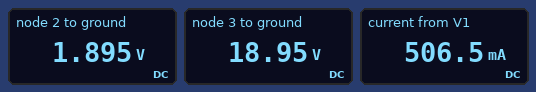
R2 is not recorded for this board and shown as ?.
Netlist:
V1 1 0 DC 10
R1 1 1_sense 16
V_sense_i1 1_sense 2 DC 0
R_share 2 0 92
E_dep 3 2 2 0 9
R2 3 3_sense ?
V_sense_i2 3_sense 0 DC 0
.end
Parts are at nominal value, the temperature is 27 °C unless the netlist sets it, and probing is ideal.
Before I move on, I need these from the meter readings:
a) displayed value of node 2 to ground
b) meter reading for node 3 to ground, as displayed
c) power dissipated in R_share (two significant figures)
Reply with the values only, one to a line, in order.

1.895 V
18.95 V
39 mW
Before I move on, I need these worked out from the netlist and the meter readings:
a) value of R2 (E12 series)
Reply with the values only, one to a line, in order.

39 Ω
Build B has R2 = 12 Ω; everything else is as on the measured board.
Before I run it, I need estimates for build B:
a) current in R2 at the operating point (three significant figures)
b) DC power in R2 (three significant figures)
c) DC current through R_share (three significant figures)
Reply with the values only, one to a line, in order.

574 mA
3.96 W
7.49 mA
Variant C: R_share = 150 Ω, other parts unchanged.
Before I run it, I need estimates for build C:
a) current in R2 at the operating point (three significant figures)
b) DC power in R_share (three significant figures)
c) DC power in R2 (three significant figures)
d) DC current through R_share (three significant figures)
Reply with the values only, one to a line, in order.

492 mA
24.6 mW
9.45 W
12.8 mA
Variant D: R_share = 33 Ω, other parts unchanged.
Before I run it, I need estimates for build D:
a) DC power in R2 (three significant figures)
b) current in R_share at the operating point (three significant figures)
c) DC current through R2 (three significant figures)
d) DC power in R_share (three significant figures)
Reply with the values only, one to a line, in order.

8.21 W
54.2 mA
459 mA
97.1 mW
